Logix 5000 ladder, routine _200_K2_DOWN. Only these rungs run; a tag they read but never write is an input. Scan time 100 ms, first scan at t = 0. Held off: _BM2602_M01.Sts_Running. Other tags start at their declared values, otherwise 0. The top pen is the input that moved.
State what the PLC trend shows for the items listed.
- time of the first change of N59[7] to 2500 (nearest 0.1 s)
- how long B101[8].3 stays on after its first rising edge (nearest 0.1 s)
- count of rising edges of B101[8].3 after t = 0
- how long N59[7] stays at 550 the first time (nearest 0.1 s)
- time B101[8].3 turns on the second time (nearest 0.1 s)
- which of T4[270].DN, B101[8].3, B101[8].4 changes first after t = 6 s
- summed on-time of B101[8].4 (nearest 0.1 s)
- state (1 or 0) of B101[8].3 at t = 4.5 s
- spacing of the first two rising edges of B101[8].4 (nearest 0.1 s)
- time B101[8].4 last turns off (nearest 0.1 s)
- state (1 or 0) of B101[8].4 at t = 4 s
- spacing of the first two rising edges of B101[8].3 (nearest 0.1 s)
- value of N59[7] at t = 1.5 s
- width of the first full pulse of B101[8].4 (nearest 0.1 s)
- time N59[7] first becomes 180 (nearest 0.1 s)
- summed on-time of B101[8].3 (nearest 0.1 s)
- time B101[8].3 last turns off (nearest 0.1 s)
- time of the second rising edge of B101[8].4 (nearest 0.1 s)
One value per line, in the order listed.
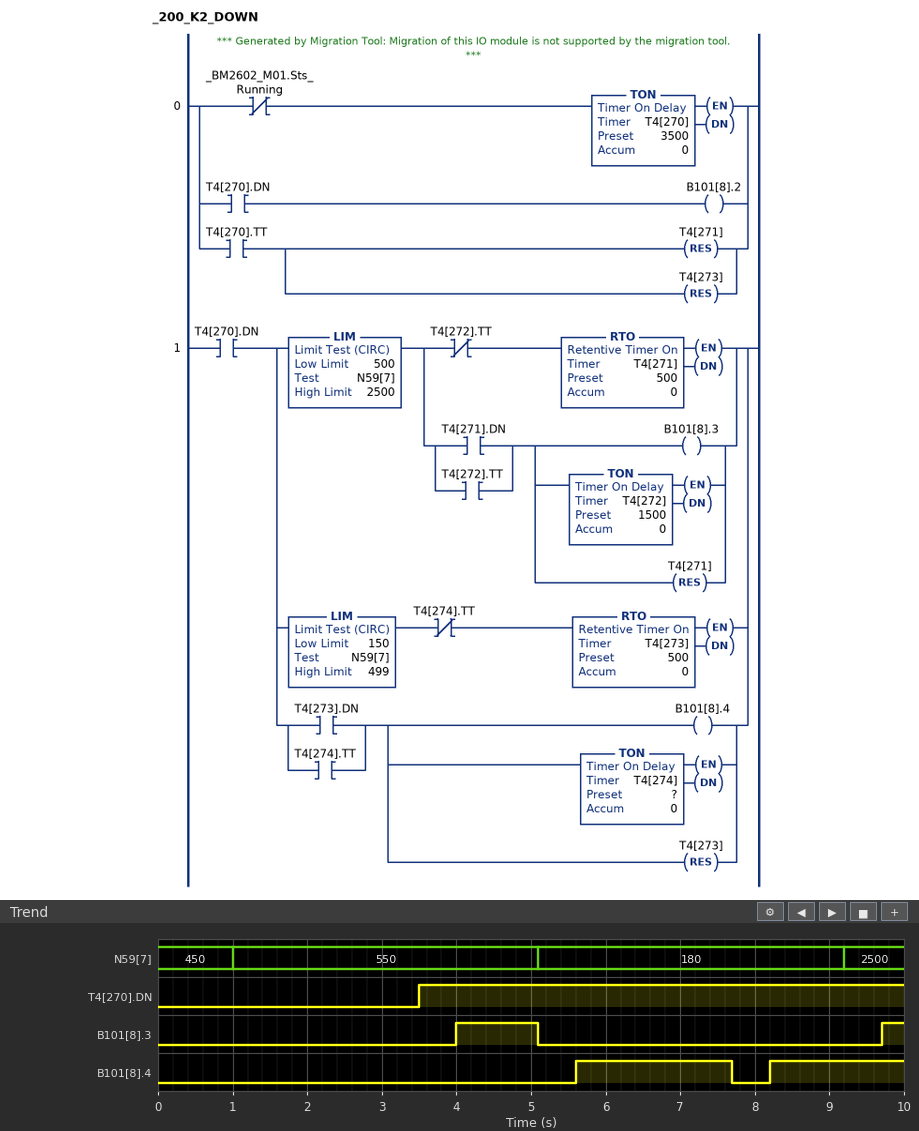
9.2 s
1.1 s
2
4.1 s
9.7 s
B101[8].4
3.9 s
1
2.6 s
7.7 s
0
5.7 s
550
2.1 s
5.1 s
1.4 s
5.1 s
8.2 s
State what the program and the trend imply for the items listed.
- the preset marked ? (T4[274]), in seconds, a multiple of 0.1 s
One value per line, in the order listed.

2.0 s
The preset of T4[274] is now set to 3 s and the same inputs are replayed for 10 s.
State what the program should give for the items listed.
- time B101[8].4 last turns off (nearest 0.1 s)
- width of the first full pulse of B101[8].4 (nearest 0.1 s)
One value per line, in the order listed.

8.7 s
3.1 s
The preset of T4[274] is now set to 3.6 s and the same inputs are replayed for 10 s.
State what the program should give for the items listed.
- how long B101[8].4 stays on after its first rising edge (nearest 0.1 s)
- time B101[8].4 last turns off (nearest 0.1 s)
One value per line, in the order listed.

3.7 s
9.3 s
